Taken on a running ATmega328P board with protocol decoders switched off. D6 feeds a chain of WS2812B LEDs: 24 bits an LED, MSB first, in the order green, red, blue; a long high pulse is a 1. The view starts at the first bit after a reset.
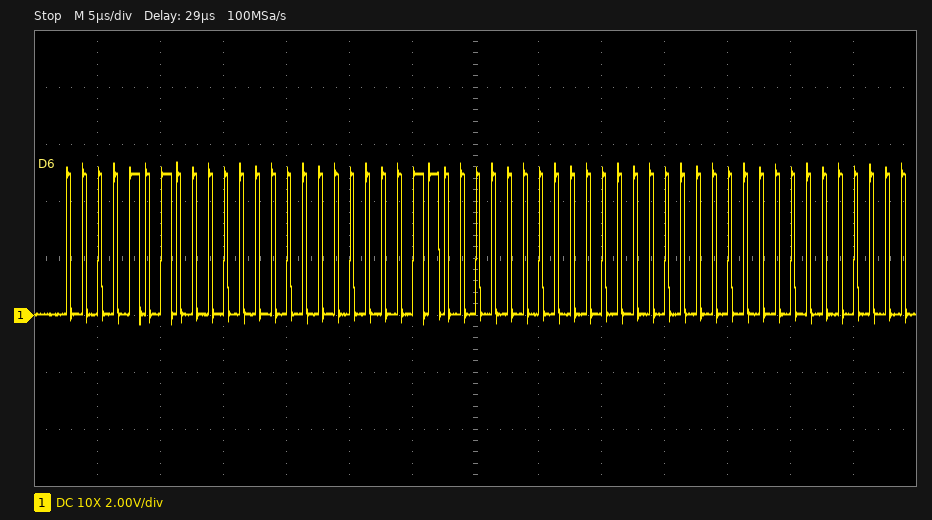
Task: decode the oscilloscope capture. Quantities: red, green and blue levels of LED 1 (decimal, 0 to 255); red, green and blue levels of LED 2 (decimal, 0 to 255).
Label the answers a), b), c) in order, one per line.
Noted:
a) 0, 10, 3
b) 0, 0, 0
